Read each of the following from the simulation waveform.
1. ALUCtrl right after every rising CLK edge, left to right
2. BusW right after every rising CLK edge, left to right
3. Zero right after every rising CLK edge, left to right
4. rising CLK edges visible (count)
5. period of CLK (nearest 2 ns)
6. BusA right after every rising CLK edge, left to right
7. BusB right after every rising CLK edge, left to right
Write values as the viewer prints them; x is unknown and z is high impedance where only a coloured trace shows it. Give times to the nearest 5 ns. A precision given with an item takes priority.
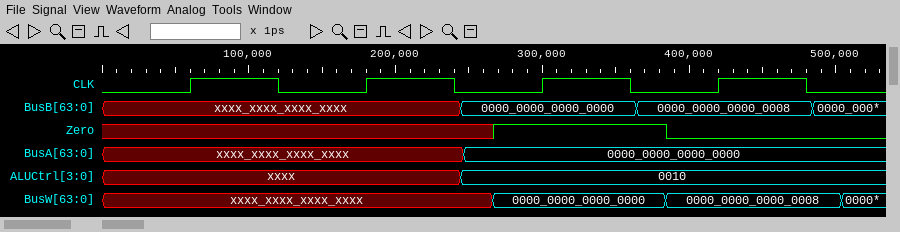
xxxx, xxxx, 0010, 0010
xxxx_xxxx_xxxx_xxxx, xxxx_xxxx_xxxx_xxxx, 0000_0000_0000_0000, 0000_0000_0000_0008
x x 1 0
4
120 ns
xxxx_xxxx_xxxx_xxxx, xxxx_xxxx_xxxx_xxxx, 0000_0000_0000_0000, 0000_0000_0000_0000
xxxx_xxxx_xxxx_xxxx, xxxx_xxxx_xxxx_xxxx, 0000_0000_0000_0000, 0000_0000_0000_0008
